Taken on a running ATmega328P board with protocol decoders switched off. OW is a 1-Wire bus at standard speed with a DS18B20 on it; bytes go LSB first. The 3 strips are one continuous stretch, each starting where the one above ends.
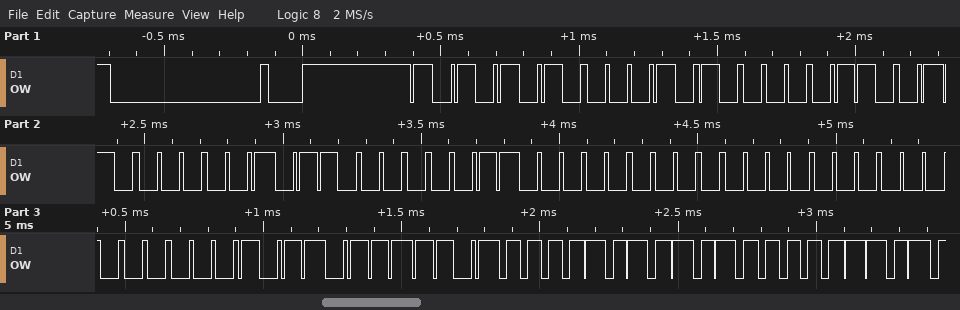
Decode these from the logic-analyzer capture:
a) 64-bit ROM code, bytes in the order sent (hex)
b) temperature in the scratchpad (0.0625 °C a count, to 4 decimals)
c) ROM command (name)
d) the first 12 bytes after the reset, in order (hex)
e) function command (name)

28 98 81 06 06 00 00 D0
85.0000 °C
Match ROM
55 28 98 81 06 06 00 00 D0 BE 50 05
Read Scratchpad
